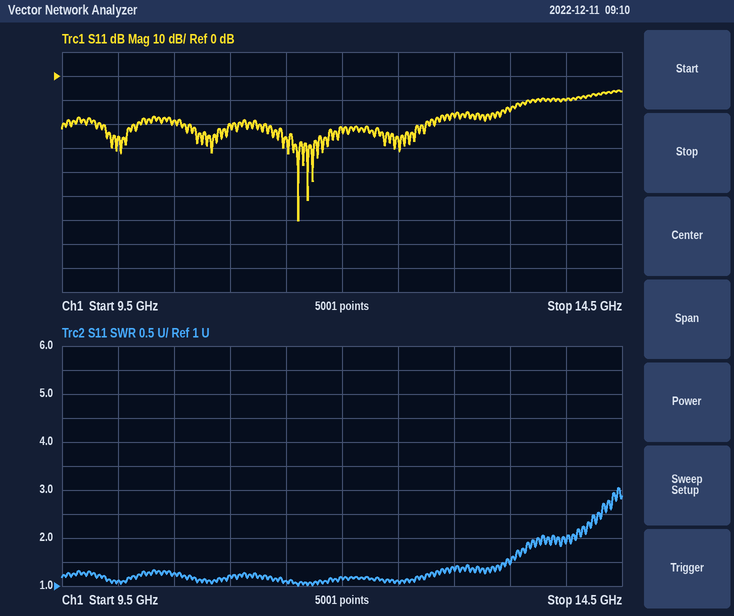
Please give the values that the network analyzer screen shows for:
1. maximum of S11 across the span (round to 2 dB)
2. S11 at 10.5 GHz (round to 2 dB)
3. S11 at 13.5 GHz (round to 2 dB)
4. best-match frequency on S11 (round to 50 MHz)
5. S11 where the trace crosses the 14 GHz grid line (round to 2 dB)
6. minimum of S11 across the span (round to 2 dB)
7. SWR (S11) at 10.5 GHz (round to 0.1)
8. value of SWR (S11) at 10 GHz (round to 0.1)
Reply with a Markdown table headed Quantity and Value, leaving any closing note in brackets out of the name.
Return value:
| Quantity | Value |
|---|---|
| maximum of S11 across the span | -6 dB |
| S11 at 10.5 GHz | -18 dB |
| S11 at 13.5 GHz | -14 dB |
| best-match frequency on S11 | 11.60 GHz |
| S11 where the trace crosses the 14 GHz grid line | -10 dB |
| minimum of S11 across the span | -60 dB |
| SWR (S11) at 10.5 GHz | 1.3 |
| value of SWR (S11) at 10 GHz | 1.1 |
